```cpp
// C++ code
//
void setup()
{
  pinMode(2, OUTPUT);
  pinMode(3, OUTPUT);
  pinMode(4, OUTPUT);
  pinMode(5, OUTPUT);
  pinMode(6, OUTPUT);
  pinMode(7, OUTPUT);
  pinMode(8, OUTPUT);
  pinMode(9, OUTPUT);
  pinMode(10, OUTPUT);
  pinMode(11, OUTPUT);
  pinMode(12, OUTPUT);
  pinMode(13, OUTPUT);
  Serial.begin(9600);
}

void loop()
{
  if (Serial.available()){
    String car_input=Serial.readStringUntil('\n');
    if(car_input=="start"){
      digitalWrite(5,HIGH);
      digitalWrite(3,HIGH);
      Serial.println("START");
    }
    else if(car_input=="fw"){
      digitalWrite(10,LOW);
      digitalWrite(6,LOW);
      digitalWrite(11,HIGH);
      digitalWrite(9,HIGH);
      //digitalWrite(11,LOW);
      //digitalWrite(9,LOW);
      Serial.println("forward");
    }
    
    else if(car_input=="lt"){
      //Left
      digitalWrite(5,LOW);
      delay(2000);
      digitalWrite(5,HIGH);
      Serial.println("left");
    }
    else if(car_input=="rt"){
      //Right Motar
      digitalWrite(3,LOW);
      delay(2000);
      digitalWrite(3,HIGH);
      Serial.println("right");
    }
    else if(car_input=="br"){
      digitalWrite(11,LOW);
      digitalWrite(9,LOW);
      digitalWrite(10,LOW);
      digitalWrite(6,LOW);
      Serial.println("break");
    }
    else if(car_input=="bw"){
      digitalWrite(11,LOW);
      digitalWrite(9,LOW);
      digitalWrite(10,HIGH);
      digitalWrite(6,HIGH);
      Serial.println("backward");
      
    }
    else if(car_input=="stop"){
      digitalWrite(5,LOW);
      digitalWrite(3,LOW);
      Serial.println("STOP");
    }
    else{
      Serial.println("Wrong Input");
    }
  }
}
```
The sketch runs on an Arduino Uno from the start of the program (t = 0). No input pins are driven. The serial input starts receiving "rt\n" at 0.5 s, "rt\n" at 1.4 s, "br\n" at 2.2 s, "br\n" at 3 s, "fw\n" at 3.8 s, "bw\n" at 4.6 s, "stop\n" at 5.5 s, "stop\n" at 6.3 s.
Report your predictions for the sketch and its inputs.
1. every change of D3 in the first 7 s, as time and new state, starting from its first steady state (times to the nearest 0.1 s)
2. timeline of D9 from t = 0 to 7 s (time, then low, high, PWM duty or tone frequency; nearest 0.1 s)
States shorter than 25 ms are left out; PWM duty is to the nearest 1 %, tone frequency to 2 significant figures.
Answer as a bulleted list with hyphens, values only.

- 0 s low; 4.5 s high; 5.5 s low
- 0 s low; 4.5 s high; 4.6 s low
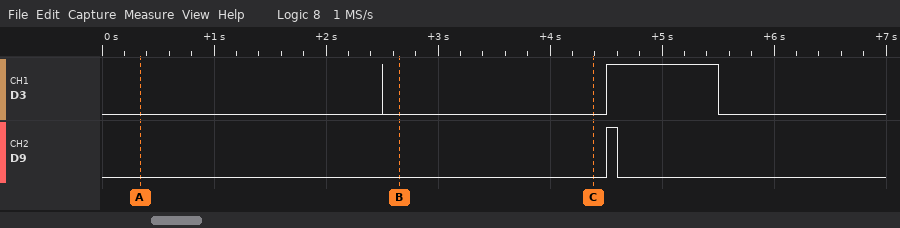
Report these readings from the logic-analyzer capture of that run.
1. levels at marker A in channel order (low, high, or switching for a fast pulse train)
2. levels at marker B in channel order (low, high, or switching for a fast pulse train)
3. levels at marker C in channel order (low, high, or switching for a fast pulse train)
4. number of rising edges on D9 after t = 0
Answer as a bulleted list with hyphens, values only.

- D3 low, D9 low
- D3 low, D9 low
- D3 low, D9 low
- 1
